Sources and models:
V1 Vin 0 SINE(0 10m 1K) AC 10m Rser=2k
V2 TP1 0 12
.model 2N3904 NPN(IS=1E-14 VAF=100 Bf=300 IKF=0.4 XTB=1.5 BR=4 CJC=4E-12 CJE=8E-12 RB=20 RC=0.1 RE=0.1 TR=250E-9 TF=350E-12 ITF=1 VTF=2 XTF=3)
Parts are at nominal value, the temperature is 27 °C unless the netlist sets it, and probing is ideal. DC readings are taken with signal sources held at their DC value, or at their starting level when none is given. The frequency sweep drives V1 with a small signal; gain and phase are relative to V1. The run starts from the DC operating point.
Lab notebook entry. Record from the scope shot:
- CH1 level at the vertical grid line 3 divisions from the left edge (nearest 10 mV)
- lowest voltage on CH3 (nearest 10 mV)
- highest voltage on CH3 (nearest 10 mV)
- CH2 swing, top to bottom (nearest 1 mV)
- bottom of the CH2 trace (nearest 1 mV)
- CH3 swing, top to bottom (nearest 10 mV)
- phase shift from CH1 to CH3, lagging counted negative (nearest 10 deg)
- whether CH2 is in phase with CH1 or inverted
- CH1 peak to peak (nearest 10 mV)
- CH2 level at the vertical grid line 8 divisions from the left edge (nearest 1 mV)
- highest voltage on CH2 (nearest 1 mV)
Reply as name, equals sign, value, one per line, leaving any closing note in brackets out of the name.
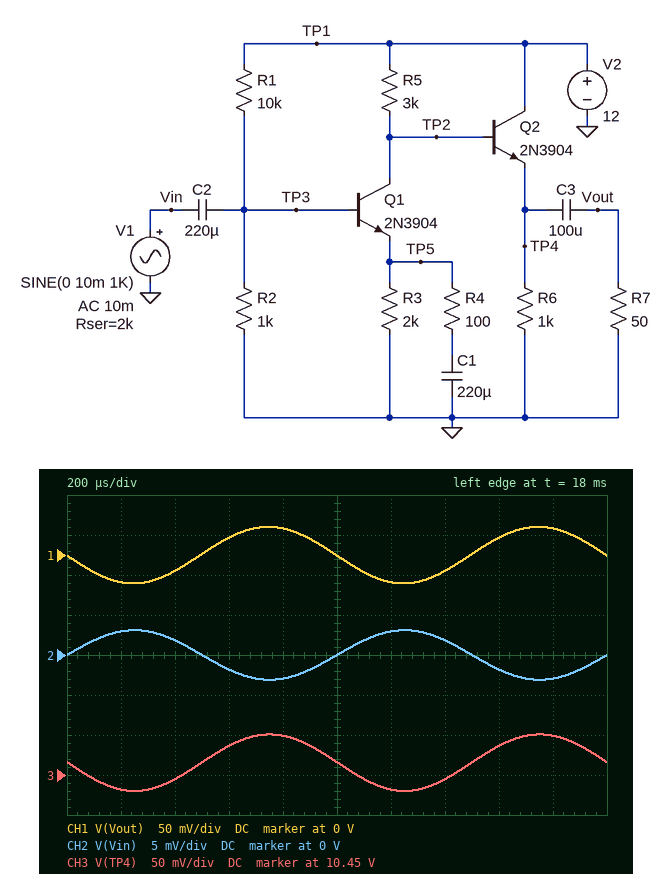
CH1 level at the vertical grid line 3 divisions from the left edge = 20 mV
lowest voltage on CH3 = 10.43 V
highest voltage on CH3 = 10.50 V
CH2 swing, top to bottom = 6 mV
bottom of the CH2 trace = -3 mV
CH3 swing, top to bottom = 70 mV
phase shift from CH1 to CH3, lagging counted negative = 0 deg
whether CH2 is in phase with CH1 or inverted = inverted
CH1 peak to peak = 70 mV
CH2 level at the vertical grid line 8 divisions from the left edge = -2 mV
highest voltage on CH2 = 3 mV
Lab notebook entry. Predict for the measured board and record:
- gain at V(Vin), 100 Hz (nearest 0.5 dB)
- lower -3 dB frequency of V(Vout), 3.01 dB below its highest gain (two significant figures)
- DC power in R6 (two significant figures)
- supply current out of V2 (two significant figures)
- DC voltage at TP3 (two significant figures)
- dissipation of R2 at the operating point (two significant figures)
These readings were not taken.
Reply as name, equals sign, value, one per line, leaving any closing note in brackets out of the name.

gain at V(Vin), 100 Hz = -10.0 dB
lower -3 dB frequency of V(Vout), 3.01 dB below its highest gain = 26 Hz
DC power in R6 = 110 mW
supply current out of V2 = 12 mA
DC voltage at TP3 = 1.1 V
dissipation of R2 at the operating point = 1.2 mW
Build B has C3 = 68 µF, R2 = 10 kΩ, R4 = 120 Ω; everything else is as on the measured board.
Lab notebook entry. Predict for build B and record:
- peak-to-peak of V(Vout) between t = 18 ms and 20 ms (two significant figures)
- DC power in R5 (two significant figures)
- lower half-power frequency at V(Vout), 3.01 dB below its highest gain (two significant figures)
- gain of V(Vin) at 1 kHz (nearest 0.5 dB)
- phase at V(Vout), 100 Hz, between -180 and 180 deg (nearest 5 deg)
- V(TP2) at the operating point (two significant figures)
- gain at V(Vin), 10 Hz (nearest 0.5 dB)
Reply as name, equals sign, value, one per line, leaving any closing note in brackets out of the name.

peak-to-peak of V(Vout) between t = 18 ms and 20 ms = 1.2 mV
DC power in R5 = 17 mW
lower half-power frequency at V(Vout), 3.01 dB below its highest gain = 41 Hz
gain of V(Vin) at 1 kHz = -21.5 dB
phase at V(Vout), 100 Hz, between -180 and 180 deg = -155 deg
V(TP2) at the operating point = 4.9 V
gain at V(Vin), 10 Hz = -19.5 dB
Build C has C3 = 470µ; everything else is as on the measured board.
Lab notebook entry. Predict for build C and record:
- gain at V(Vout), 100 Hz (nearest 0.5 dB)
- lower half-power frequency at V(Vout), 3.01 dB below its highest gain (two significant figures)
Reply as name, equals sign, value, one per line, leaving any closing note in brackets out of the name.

gain at V(Vout), 100 Hz = 11.0 dB
lower half-power frequency at V(Vout), 3.01 dB below its highest gain = 7.0 Hz
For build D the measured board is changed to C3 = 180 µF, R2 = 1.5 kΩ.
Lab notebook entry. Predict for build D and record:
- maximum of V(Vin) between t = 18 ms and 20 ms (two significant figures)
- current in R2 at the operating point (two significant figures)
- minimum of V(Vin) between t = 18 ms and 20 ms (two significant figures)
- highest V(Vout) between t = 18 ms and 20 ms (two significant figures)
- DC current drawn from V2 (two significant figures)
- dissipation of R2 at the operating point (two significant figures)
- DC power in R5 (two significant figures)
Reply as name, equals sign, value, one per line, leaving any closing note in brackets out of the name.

maximum of V(Vin) between t = 18 ms and 20 ms = 3.9 mV
current in R2 at the operating point = 1.0 mA
minimum of V(Vin) between t = 18 ms and 20 ms = -3.9 mV
highest V(Vout) between t = 18 ms and 20 ms = 60 mV
DC current drawn from V2 = 11 mA
dissipation of R2 at the operating point = 1.6 mW
DC power in R5 = 740 µW
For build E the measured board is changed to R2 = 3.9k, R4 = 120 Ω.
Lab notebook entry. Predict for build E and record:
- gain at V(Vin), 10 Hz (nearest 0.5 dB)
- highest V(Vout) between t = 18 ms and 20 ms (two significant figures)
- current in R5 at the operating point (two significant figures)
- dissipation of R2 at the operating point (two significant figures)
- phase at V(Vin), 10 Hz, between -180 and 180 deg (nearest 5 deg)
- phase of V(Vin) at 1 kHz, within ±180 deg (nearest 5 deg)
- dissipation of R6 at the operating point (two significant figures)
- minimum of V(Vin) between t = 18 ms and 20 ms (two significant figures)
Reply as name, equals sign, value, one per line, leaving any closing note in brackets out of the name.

gain at V(Vin), 10 Hz = -5.0 dB
highest V(Vout) between t = 18 ms and 20 ms = 99 mV
current in R5 at the operating point = 1.4 mA
dissipation of R2 at the operating point = 2.9 mW
phase at V(Vin), 10 Hz, between -180 and 180 deg = 0 deg
phase of V(Vin) at 1 kHz, within ±180 deg = 0 deg
dissipation of R6 at the operating point = 52 mW
minimum of V(Vin) between t = 18 ms and 20 ms = -5.7 mV
